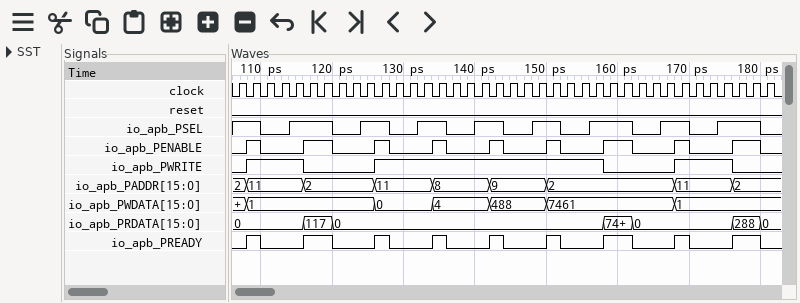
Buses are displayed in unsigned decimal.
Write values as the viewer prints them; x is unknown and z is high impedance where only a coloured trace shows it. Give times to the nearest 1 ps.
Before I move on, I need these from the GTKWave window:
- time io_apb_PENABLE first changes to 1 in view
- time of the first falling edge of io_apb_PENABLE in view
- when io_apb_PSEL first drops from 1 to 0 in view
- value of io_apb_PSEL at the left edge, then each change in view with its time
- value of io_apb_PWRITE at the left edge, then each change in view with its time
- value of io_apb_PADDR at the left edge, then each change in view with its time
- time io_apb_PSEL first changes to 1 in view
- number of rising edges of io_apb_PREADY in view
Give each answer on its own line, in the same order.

108 ps
110 ps
110 ps
1, 0 at 110 ps, 1 at 114 ps, 0 at 120 ps, 1 at 124 ps, 0 at 128 ps, 1 at 132 ps, 0 at 136 ps, 1 at 140 ps, 0 at 144 ps, 1 at 148 ps, 0 at 152 ps, 1 at 156 ps, 0 at 162 ps, 1 at 166 ps, 0 at 170 ps, 1 at 174 ps, 0 at 180 ps
0, 1 at 108 ps, 0 at 116 ps, 1 at 126 ps, 0 at 158 ps, 1 at 168 ps, 0 at 176 ps
2, 11 at 108 ps, 2 at 116 ps, 11 at 126 ps, 8 at 134 ps, 9 at 142 ps, 2 at 150 ps, 11 at 168 ps, 2 at 176 ps
114 ps
9
